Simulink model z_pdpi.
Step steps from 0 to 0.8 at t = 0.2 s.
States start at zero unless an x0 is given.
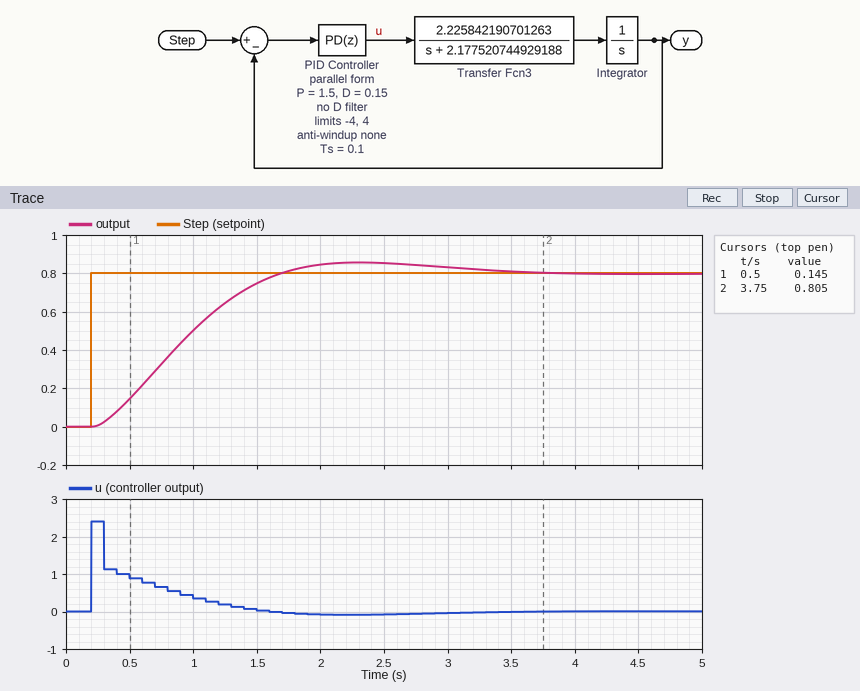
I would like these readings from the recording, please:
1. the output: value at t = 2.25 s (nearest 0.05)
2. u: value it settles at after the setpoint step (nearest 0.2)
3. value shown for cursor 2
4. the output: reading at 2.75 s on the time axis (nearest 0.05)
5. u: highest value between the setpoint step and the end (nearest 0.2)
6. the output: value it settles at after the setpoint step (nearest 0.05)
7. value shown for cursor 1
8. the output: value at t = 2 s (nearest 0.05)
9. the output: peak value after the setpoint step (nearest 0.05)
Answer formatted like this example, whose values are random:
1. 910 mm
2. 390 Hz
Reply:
1. 0.85
2. 0.0
3. 0.805
4. 0.85
5. 2.4
6. 0.80
7. 0.145
8. 0.85
9. 0.85
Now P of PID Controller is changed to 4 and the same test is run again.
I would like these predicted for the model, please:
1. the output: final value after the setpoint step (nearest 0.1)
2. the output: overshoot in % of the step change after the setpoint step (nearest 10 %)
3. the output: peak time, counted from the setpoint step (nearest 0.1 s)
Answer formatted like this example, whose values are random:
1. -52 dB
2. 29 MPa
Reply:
1. 0.8
2. 30 %
3. 1.1 s
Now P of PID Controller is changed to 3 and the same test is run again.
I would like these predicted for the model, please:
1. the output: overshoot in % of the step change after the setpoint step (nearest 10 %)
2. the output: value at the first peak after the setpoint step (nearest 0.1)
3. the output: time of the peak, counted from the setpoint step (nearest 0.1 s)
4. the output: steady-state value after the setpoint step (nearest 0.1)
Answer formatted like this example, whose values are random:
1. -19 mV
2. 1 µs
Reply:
1. 20 %
2. 1.0
3. 1.3 s
4. 0.8
